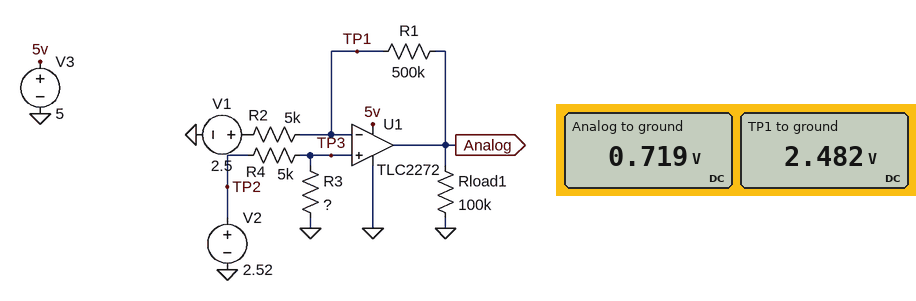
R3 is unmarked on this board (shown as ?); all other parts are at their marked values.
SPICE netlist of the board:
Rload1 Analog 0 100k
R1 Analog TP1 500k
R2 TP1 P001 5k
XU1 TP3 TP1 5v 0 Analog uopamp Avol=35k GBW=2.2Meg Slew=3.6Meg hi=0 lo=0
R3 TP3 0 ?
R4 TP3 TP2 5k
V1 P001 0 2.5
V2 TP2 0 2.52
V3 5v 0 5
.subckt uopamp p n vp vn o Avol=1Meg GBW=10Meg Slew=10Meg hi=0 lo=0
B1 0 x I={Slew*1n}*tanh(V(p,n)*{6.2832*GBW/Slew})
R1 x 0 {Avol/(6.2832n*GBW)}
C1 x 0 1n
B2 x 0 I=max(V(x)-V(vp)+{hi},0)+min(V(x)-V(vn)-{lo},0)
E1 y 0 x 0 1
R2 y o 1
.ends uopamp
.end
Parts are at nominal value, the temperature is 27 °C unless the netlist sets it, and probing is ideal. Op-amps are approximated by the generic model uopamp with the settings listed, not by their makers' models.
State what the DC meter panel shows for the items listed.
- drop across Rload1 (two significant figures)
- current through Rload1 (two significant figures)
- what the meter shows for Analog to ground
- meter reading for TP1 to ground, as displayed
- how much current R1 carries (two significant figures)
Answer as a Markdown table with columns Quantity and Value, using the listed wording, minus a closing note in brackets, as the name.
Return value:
| Quantity | Value |
|---|---|
| drop across Rload1 | 720 mV |
| current through Rload1 | 7.2 µA |
| what the meter shows for Analog to ground | 0.719 V |
| meter reading for TP1 to ground, as displayed | 2.482 V |
| how much current R1 carries | 3.5 µA |
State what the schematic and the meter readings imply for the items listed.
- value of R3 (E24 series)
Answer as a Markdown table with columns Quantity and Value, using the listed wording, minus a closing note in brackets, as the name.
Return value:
| Quantity | Value |
|---|---|
| value of R3 | 330 kΩ |
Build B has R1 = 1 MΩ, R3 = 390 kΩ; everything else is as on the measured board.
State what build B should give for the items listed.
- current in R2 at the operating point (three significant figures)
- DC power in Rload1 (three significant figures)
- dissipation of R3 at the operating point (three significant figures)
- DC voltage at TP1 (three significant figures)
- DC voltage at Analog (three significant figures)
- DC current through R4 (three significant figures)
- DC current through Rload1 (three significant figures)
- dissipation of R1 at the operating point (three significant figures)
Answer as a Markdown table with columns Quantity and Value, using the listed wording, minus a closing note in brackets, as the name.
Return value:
| Quantity | Value |
|---|---|
| current in R2 at the operating point | 2.38 µA |
| DC power in Rload1 | 116 nW |
| dissipation of R3 at the operating point | 15.9 µW |
| DC voltage at TP1 | 2.49 V |
| DC voltage at Analog | 108 mV |
| DC current through R4 | 6.38 µA |
| DC current through Rload1 | 1.08 µA |
| dissipation of R1 at the operating point | 5.67 µW |
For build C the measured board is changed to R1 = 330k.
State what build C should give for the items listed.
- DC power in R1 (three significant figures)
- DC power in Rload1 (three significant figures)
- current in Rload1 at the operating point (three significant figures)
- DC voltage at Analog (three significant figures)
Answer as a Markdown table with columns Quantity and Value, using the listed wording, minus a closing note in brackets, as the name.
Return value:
| Quantity | Value |
|---|---|
| DC power in R1 | 4.11 µW |
| DC power in Rload1 | 17.4 µW |
| current in Rload1 at the operating point | 13.2 µA |
| DC voltage at Analog | 1.32 V |
